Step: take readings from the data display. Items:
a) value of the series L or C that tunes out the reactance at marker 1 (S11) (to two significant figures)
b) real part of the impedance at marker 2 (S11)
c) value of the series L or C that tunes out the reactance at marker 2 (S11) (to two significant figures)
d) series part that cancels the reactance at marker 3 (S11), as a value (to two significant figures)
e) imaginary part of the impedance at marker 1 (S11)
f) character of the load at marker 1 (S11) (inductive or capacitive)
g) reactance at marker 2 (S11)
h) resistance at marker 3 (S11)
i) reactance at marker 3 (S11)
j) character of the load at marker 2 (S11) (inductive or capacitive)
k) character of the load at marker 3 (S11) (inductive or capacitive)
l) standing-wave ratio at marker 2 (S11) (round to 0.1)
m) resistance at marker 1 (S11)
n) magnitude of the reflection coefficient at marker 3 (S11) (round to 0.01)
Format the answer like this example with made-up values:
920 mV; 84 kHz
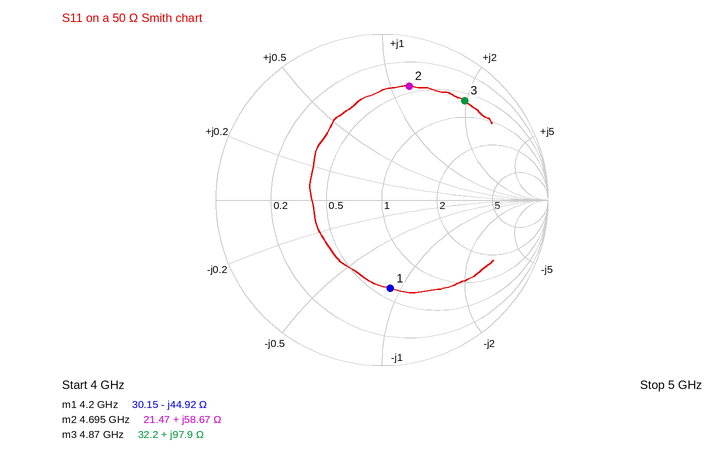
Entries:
1.7 nH; 21.47 Ω; 580 fF; 330 fF; -44.92 Ω; capacitive; +58.67 Ω; 32.2 Ω; +97.9 Ω; inductive; inductive; 5.8; 30.15 Ω; 0.78
